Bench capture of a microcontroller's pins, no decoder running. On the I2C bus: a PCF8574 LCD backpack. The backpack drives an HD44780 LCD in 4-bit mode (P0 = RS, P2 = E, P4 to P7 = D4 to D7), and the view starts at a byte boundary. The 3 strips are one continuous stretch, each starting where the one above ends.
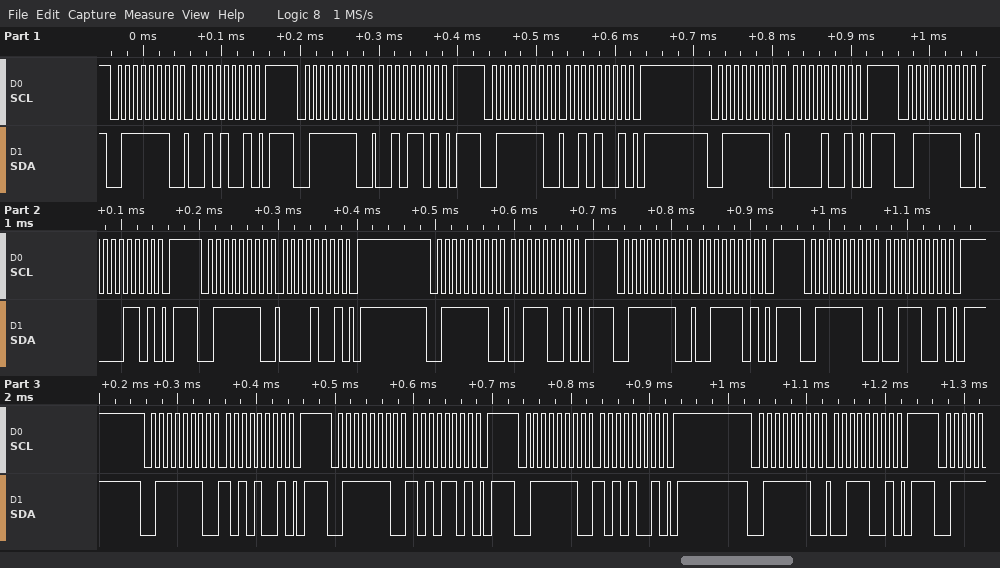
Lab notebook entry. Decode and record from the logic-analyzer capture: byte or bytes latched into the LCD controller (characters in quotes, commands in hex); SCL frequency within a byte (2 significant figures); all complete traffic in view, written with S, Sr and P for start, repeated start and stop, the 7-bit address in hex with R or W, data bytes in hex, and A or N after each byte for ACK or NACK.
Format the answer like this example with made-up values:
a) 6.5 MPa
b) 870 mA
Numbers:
a) ' ' ':'
b) 100 kHz
c) S 3FW A 29 A P S 3FW A 2D A P S 3FW A 29 A P S 3FW A 09 A P S 3FW A 0D A P S 3FW A 09 A P S 3FW A 39 A P S 3FW A 3D A P S 3FW A 39 A P S 3FW A A9 A P S 3FW A AD A P S 3FW A A9 A P S 3FW A 39 A P
